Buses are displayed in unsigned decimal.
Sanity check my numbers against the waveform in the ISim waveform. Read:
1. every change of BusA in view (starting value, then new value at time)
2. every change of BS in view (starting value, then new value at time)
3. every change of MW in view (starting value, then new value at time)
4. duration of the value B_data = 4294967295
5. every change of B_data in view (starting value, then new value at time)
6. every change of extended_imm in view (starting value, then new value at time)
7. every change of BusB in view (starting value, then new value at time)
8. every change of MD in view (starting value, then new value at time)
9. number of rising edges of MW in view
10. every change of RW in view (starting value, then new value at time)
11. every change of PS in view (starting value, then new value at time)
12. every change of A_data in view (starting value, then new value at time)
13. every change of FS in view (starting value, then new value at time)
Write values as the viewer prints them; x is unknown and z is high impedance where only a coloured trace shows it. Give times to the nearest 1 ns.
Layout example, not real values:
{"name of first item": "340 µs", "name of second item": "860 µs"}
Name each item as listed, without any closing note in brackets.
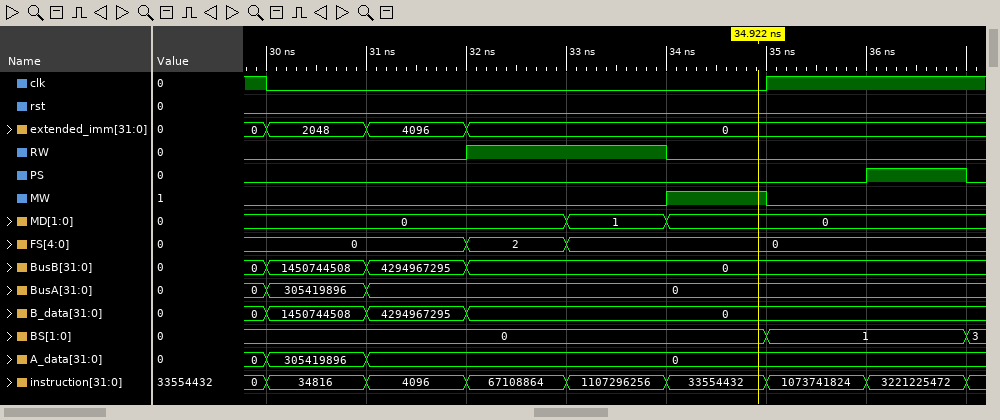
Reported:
{"every change of BusA in view": "0, 305419896 at 30 ns, 0 at 31 ns", "every change of BS in view": "0, 1 at 35 ns, 3 at 37 ns", "every change of MW in view": "0, 1 at 34 ns, 0 at 35 ns", "duration of the value B_data = 4294967295": "1 ns", "every change of B_data in view": "0, 1450744508 at 30 ns, 4294967295 at 31 ns, 0 at 32 ns", "every change of extended_imm in view": "0, 2048 at 30 ns, 4096 at 31 ns, 0 at 32 ns", "every change of BusB in view": "0, 1450744508 at 30 ns, 4294967295 at 31 ns, 0 at 32 ns", "every change of MD in view": "0, 1 at 33 ns, 0 at 34 ns", "number of rising edges of MW in view": "1", "every change of RW in view": "0, 1 at 32 ns, 0 at 34 ns", "every change of PS in view": "0, 1 at 36 ns, 0 at 37 ns", "every change of A_data in view": "0, 305419896 at 30 ns, 0 at 31 ns", "every change of FS in view": "0, 2 at 32 ns, 0 at 33 ns"}
